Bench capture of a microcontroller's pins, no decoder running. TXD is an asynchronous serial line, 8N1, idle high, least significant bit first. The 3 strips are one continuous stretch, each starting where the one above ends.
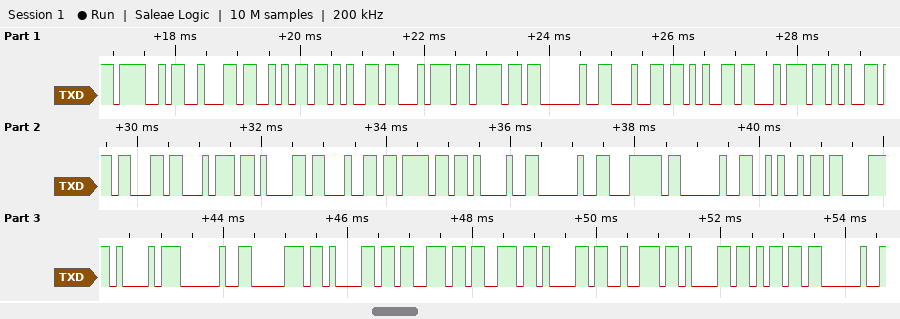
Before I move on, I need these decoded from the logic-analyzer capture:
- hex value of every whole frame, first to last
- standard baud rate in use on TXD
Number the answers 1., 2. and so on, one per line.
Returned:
1. 0x4F 0x62 0x6A 0x65 0x74 0x6F 0x20 0x64 0x65 0x74 0x65 0x63 0x74 0x61 0x64 0x6F 0x21 0x20 0x7C 0x20 0x4A 0xC3 0xA1 0x20 0x70 0x61 0x73 0x73 0x61 0x72 0x61 0x6D 0x20
2. 9600 baud
